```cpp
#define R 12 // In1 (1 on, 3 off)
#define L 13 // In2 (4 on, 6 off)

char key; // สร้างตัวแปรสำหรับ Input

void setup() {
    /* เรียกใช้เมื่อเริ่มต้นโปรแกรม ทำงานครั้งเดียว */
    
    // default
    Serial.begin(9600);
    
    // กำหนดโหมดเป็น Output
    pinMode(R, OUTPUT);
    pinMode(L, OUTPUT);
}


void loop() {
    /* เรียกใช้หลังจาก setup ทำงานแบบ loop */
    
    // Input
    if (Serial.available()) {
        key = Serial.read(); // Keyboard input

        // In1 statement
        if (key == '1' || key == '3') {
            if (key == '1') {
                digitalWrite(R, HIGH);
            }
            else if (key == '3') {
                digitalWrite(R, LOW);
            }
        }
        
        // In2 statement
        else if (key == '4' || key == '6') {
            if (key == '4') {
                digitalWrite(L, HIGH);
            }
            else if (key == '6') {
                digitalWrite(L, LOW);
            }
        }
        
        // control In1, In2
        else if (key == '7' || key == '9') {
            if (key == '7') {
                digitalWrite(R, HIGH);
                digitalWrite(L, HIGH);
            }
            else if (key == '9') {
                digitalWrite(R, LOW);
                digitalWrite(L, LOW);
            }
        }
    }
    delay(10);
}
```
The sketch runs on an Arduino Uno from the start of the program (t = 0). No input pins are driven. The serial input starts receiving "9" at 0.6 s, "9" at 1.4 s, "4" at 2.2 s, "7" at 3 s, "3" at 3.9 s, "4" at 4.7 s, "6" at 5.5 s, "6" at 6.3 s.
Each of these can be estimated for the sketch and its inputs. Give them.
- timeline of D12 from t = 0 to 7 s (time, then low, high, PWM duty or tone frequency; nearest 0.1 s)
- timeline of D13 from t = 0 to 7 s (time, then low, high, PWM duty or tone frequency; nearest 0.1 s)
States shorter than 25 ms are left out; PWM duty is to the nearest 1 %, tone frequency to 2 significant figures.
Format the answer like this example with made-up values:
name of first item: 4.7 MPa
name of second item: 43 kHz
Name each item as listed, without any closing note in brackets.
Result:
timeline of D12 from t = 0 to 7 s: 0 s low; 3 s high; 3.9 s low
timeline of D13 from t = 0 to 7 s: 0 s low; 2.2 s high; 5.5 s low
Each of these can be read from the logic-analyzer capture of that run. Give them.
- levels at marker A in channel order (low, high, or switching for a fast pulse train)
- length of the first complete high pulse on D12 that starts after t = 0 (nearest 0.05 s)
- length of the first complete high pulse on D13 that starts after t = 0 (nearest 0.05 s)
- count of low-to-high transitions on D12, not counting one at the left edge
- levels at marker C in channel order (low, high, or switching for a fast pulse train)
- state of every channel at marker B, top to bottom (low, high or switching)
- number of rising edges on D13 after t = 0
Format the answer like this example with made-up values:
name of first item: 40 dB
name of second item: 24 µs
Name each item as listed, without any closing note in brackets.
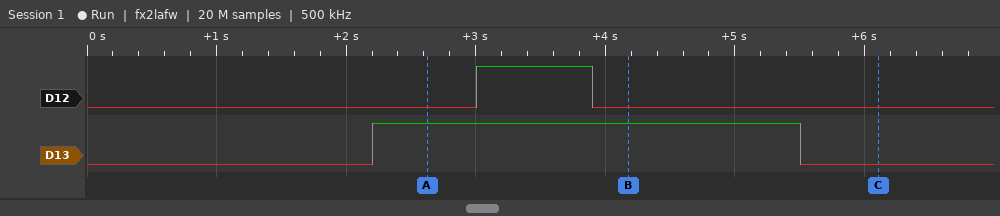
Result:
levels at marker A in channel order: D12 low, D13 high
length of the first complete high pulse on D12 that starts after t = 0: 0.90 s
length of the first complete high pulse on D13 that starts after t = 0: 3.30 s
count of low-to-high transitions on D12, not counting one at the left edge: 1
levels at marker C in channel order: D12 low, D13 low
state of every channel at marker B, top to bottom: D12 low, D13 high
number of rising edges on D13 after t = 0: 1
